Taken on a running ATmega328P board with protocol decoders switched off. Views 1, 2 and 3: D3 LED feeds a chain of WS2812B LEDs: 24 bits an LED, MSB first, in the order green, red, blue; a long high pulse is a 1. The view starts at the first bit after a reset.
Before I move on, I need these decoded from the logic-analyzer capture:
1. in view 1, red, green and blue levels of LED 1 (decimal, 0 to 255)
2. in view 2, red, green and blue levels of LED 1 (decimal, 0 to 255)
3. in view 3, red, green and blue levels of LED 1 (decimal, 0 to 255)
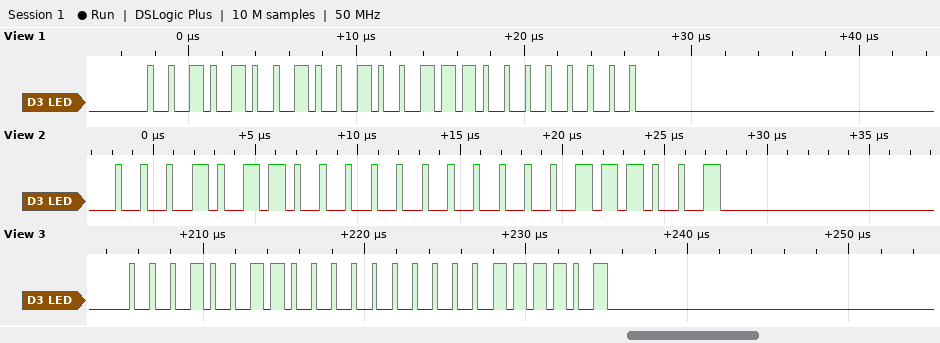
39, 41, 0
0, 22, 57
0, 19, 61
